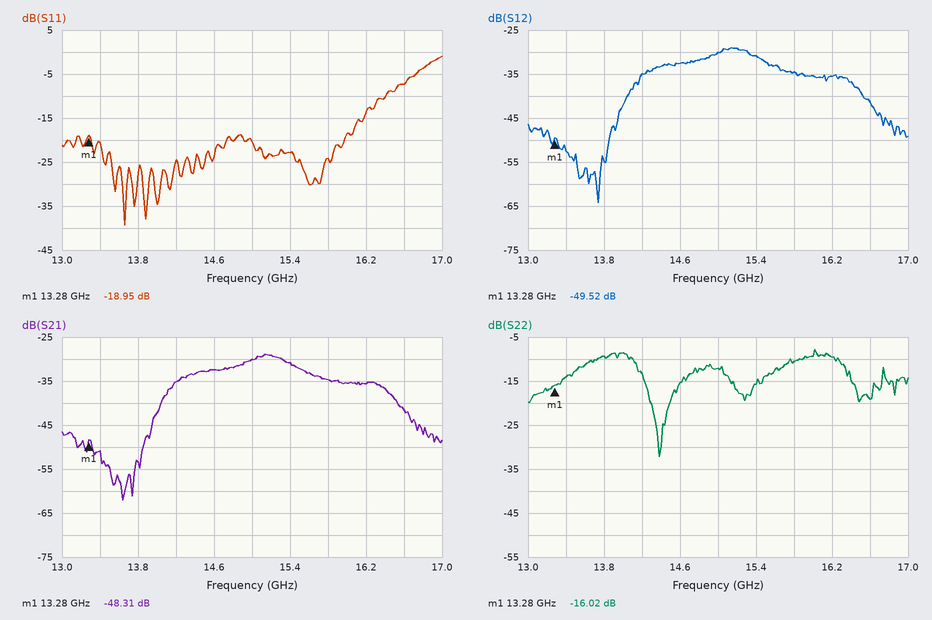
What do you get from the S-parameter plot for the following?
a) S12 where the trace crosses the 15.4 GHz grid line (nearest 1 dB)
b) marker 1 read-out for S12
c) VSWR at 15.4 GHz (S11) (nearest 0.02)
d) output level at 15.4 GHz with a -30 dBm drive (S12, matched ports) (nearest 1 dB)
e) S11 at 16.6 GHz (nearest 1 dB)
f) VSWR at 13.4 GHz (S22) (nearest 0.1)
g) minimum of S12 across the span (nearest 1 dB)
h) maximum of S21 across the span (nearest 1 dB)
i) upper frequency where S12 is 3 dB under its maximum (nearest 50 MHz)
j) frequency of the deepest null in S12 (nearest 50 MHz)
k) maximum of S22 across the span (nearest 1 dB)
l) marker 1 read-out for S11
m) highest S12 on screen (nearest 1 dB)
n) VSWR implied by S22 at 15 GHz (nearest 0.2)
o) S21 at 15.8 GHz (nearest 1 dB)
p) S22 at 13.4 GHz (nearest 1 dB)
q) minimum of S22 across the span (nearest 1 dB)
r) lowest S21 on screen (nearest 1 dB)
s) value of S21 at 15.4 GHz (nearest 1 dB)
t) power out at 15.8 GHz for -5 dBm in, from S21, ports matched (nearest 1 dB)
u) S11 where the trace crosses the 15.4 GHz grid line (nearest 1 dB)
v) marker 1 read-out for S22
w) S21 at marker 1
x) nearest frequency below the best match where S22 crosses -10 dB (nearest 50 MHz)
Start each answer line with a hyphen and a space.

- -31 dB
- -49.52 dB
- 1.16
- -61 dBm
- -7 dB
- 1.5
- -64 dB
- -29 dB
- 15.50 GHz
- 13.75 GHz
- -8 dB
- -18.95 dB
- -29 dB
- 1.6
- -35 dB
- -14 dB
- -32 dB
- -62 dB
- -31 dB
- -40 dBm
- -23 dB
- -16.02 dB
- -48.31 dB
- 14.10 GHz
